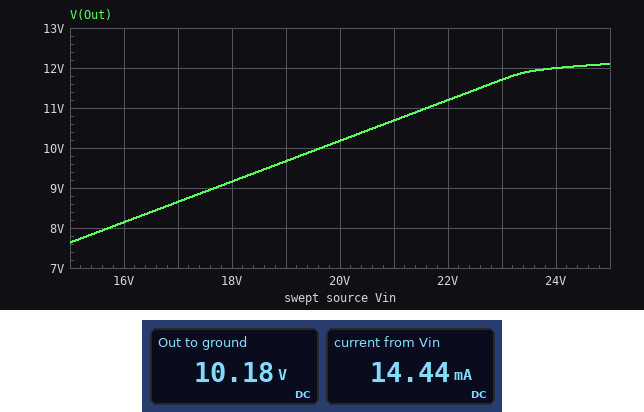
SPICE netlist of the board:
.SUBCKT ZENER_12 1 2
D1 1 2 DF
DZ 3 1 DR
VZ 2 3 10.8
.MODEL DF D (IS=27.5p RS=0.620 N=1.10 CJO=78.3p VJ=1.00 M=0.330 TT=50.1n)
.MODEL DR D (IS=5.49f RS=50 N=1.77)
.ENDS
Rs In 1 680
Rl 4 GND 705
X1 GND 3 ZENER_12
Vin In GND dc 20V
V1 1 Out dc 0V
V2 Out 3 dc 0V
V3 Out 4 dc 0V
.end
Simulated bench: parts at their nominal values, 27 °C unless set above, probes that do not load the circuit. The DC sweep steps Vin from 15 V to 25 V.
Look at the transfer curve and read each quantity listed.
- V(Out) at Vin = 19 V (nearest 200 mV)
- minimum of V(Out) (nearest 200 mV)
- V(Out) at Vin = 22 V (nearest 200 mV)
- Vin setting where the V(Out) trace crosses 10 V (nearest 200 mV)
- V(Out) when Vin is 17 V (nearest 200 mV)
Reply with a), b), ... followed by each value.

a) 9.6 V
b) 7.6 V
c) 11.2 V
d) 19.6 V
e) 8.6 V
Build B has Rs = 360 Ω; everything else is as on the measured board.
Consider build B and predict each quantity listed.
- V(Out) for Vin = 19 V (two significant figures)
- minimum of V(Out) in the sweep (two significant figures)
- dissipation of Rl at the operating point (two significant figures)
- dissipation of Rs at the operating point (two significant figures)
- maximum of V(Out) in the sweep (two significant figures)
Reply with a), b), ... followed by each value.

a) 12 V
b) 9.9 V
c) 210 mW
d) 170 mW
e) 13 V
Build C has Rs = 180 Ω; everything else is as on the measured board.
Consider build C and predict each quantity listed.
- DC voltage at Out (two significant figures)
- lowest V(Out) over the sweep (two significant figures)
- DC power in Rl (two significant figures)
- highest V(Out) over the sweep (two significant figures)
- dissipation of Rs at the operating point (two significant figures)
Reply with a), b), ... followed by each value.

a) 13 V
b) 12 V
c) 240 mW
d) 14 V
e) 260 mW
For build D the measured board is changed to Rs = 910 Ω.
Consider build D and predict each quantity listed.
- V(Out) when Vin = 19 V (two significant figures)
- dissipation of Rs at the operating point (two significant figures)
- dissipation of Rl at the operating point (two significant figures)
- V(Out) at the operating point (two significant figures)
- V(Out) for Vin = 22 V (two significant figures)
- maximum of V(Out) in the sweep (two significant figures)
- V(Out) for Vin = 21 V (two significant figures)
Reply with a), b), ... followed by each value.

a) 8.3 V
b) 140 mW
c) 110 mW
d) 8.7 V
e) 9.6 V
f) 11 V
g) 9.2 V
